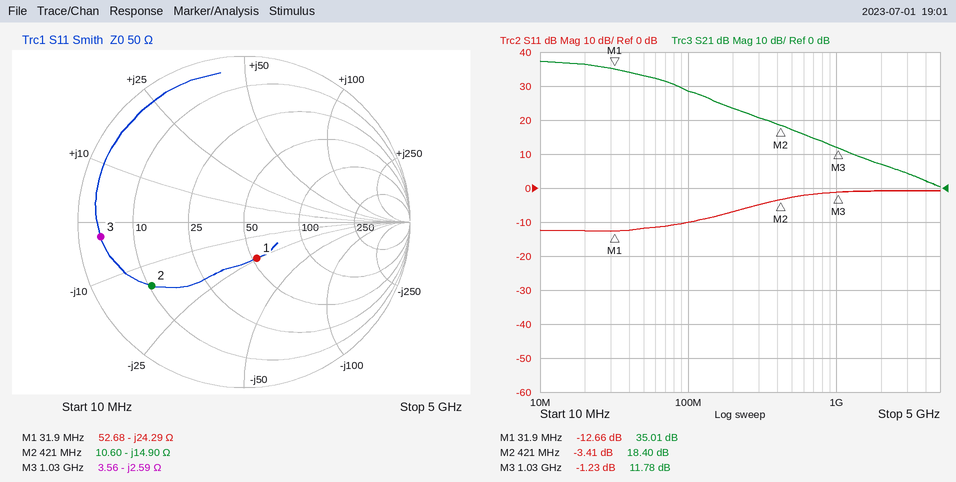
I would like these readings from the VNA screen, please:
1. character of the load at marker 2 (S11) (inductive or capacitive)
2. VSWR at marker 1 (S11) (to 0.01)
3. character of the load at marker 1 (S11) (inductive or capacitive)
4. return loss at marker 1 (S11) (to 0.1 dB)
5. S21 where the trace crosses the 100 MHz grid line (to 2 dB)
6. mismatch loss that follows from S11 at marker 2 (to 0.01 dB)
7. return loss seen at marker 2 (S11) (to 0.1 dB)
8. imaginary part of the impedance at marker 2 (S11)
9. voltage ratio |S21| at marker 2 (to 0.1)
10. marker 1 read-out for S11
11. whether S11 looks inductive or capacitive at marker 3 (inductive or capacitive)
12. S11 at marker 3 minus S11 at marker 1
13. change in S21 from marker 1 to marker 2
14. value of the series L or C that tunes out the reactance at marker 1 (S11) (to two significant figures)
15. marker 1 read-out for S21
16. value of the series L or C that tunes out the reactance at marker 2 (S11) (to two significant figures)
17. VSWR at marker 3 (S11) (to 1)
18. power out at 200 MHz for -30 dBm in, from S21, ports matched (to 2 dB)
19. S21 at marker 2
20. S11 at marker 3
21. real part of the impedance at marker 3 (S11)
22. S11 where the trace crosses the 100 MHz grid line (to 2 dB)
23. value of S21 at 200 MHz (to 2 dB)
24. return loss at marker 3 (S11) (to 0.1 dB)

capacitive
1.61
capacitive
12.7 dB
28 dB
2.64 dB
3.4 dB
-14.90 Ω
8.3
-12.66 dB
capacitive
11.43 dB
-16.61 dB
120 nH
35.01 dB
5.6 nH
14
-6 dBm
18.40 dB
-1.23 dB
3.56 Ω
-10 dB
24 dB
1.2 dB
